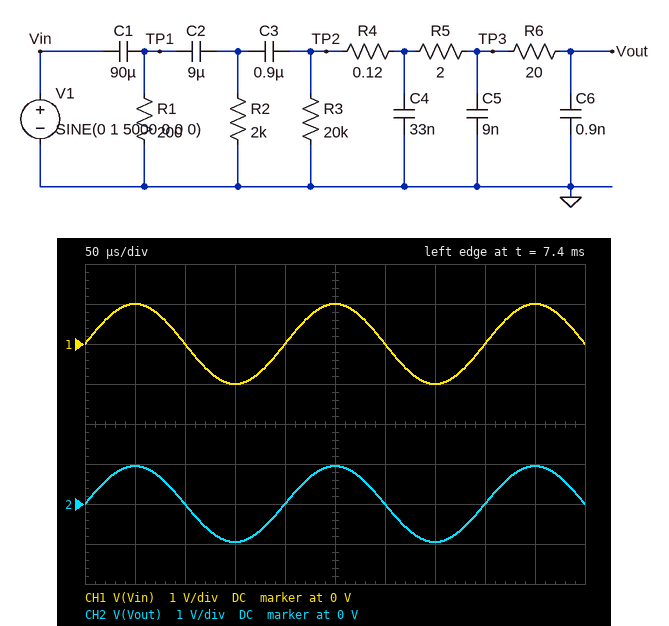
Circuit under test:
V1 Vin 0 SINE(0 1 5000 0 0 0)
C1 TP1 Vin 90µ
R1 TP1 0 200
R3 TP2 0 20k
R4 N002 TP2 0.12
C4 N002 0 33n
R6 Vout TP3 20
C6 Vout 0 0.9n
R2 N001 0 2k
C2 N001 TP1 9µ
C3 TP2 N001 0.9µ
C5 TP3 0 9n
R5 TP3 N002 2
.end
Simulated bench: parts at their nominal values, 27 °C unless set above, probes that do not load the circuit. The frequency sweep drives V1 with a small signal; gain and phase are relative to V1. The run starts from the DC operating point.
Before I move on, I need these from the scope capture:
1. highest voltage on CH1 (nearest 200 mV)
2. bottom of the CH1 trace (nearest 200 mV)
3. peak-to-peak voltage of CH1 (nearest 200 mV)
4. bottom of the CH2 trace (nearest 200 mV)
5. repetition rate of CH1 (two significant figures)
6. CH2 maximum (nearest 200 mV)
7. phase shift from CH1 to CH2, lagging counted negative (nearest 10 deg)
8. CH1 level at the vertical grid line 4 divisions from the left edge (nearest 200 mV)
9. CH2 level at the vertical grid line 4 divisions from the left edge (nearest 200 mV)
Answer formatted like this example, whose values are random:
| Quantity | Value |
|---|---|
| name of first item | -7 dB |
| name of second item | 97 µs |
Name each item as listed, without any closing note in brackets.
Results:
| Quantity | Value |
|---|---|
| highest voltage on CH1 | 1.0 V |
| bottom of the CH1 trace | -1.0 V |
| peak-to-peak voltage of CH1 | 2.0 V |
| bottom of the CH2 trace | -1.0 V |
| repetition rate of CH1 | 5.0 kHz |
| CH2 maximum | 1.0 V |
| phase shift from CH1 to CH2, lagging counted negative | 0 deg |
| CH1 level at the vertical grid line 4 divisions from the left edge | 0 V |
| CH2 level at the vertical grid line 4 divisions from the left edge | 0 V |
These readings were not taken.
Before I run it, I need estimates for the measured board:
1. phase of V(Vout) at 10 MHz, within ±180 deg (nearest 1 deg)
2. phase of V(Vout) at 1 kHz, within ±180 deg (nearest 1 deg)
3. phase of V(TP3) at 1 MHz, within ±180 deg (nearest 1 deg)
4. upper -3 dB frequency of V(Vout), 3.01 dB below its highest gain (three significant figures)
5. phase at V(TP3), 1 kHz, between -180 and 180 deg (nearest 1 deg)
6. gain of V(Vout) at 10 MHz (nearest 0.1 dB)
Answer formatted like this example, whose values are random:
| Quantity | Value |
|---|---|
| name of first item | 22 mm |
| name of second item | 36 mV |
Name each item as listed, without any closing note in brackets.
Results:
| Quantity | Value |
|---|---|
| phase of V(Vout) at 10 MHz, within ±180 deg | -111 deg |
| phase of V(Vout) at 1 kHz, within ±180 deg | 2 deg |
| phase of V(TP3) at 1 MHz, within ±180 deg | -9 deg |
| upper -3 dB frequency of V(Vout), 3.01 dB below its highest gain | 5.10 MHz |
| phase at V(TP3), 1 kHz, between -180 and 180 deg | 2 deg |
| gain of V(Vout) at 10 MHz | -8.5 dB |
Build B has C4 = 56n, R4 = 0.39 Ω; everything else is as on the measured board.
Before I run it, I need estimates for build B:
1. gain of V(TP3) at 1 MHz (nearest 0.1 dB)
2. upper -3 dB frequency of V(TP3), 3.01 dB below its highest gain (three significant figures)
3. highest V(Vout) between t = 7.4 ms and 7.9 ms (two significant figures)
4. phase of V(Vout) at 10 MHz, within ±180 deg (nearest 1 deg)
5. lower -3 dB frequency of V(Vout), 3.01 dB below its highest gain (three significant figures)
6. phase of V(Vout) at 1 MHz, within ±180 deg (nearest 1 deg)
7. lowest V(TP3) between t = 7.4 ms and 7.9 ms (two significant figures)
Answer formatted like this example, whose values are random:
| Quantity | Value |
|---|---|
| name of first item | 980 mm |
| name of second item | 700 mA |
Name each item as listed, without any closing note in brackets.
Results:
| Quantity | Value |
|---|---|
| gain of V(TP3) at 1 MHz | -0.9 dB |
| upper -3 dB frequency of V(TP3), 3.01 dB below its highest gain | 4.49 MHz |
| highest V(Vout) between t = 7.4 ms and 7.9 ms | 920 mV |
| phase of V(Vout) at 10 MHz, within ±180 deg | -148 deg |
| lower -3 dB frequency of V(Vout), 3.01 dB below its highest gain | 18.7 Hz |
| phase of V(Vout) at 1 MHz, within ±180 deg | -22 deg |
| lowest V(TP3) between t = 7.4 ms and 7.9 ms | -930 mV |
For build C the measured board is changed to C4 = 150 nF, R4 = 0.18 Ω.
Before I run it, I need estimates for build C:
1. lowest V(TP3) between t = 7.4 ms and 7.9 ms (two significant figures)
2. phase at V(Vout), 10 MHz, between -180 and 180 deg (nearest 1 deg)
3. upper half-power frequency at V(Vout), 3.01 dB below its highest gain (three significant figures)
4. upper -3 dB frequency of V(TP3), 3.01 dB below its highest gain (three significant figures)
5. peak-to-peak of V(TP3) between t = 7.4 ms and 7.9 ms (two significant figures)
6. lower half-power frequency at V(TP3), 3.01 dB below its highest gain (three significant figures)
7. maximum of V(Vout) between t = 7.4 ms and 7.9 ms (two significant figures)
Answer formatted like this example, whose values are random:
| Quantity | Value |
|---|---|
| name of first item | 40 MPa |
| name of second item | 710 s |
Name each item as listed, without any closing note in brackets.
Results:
| Quantity | Value |
|---|---|
| lowest V(TP3) between t = 7.4 ms and 7.9 ms | -840 mV |
| phase at V(Vout), 10 MHz, between -180 and 180 deg | -151 deg |
| upper half-power frequency at V(Vout), 3.01 dB below its highest gain | 3.83 MHz |
| upper -3 dB frequency of V(TP3), 3.01 dB below its highest gain | 4.55 MHz |
| peak-to-peak of V(TP3) between t = 7.4 ms and 7.9 ms | 1.7 V |
| lower half-power frequency at V(TP3), 3.01 dB below its highest gain | 18.0 Hz |
| maximum of V(Vout) between t = 7.4 ms and 7.9 ms | 830 mV |
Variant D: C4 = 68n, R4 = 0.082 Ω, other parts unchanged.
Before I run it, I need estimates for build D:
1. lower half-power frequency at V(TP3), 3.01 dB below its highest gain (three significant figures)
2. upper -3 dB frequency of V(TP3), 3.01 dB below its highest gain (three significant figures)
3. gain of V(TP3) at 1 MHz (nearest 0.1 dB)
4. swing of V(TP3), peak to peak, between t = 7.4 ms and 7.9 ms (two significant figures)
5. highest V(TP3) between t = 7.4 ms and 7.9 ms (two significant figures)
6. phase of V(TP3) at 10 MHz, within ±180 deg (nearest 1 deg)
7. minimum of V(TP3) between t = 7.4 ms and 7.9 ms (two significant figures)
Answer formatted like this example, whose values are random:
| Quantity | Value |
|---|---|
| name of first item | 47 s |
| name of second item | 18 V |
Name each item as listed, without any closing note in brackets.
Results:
| Quantity | Value |
|---|---|
| lower half-power frequency at V(TP3), 3.01 dB below its highest gain | 18.6 Hz |
| upper -3 dB frequency of V(TP3), 3.01 dB below its highest gain | 7.30 MHz |
| gain of V(TP3) at 1 MHz | -0.9 dB |
| swing of V(TP3), peak to peak, between t = 7.4 ms and 7.9 ms | 1.8 V |
| highest V(TP3) between t = 7.4 ms and 7.9 ms | 910 mV |
| phase of V(TP3) at 10 MHz, within ±180 deg | -66 deg |
| minimum of V(TP3) between t = 7.4 ms and 7.9 ms | -910 mV |
